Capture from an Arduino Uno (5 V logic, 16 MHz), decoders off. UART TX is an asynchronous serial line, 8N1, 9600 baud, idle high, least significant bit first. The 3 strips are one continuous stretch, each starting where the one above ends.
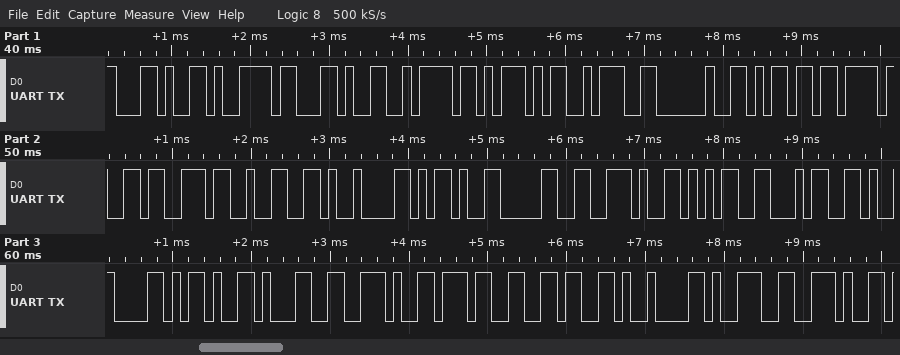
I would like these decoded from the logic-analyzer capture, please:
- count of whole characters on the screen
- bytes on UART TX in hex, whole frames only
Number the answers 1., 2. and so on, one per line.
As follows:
1. 26
2. 0x2C 0x79 0x2C 0x7A 0x5D 0x3A 0x20 0x6D 0x2F 0x73 0x32 0x09 0x2D 0x30 0x2E 0x35 0x34 0x09 0x2D 0x31 0x2E 0x37 0x36 0x09 0x39 0x2E
